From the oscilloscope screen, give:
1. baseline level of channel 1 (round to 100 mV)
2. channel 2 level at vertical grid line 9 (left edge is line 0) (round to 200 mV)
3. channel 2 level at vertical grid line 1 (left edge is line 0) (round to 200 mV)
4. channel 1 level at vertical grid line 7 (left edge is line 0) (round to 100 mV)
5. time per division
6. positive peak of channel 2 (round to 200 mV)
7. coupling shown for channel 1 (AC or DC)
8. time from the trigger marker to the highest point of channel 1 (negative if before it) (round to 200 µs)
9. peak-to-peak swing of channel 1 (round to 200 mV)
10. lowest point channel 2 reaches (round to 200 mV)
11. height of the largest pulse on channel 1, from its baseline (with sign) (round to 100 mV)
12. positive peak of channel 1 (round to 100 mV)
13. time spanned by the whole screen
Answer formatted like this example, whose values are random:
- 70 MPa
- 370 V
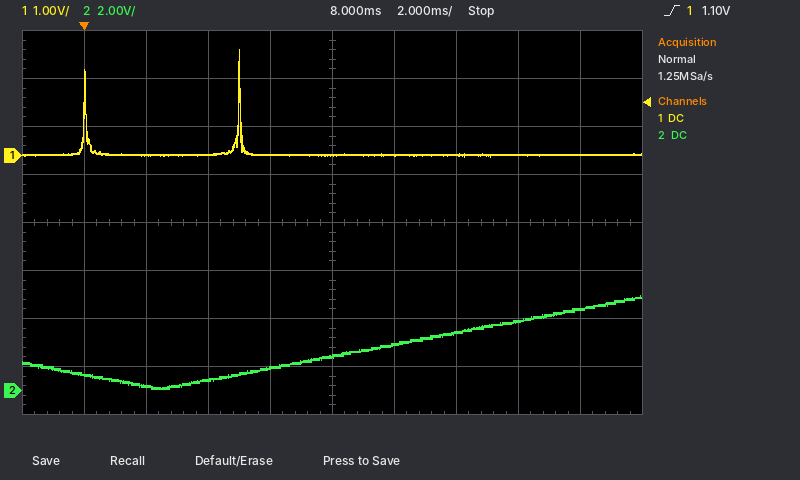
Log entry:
- 0.0 V
- 3.4 V
- 600 mV
- 0.0 V
- 2 ms
- 4.0 V
- DC
- +5.0 ms
- 2.2 V
- 0.0 V
- +2.2 V
- 2.2 V
- 20 ms
